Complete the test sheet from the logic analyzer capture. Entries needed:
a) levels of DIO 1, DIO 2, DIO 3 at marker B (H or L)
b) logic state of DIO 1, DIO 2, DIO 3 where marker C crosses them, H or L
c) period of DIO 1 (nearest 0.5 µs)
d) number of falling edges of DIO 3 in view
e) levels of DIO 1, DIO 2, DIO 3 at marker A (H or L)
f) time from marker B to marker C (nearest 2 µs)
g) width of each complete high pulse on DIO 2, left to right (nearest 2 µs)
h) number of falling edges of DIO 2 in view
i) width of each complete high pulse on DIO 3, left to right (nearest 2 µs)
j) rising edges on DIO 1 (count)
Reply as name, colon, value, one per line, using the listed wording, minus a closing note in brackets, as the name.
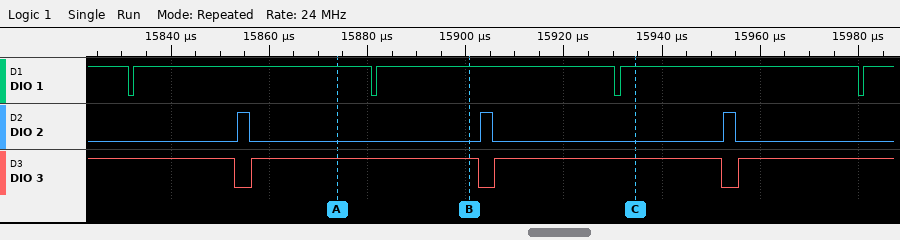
levels of DIO 1, DIO 2, DIO 3 at marker B: DIO 1=H, DIO 2=L, DIO 3=H
logic state of DIO 1, DIO 2, DIO 3 where marker C crosses them, H or L: DIO 1=H, DIO 2=L, DIO 3=H
period of DIO 1: 49.5 µs
number of falling edges of DIO 3 in view: 3
levels of DIO 1, DIO 2, DIO 3 at marker A: DIO 1=H, DIO 2=L, DIO 3=H
time from marker B to marker C: 34 µs
width of each complete high pulse on DIO 2, left to right: 2 µs, 2 µs, 2 µs
number of falling edges of DIO 2 in view: 3
width of each complete high pulse on DIO 3, left to right: 46 µs, 46 µs
rising edges on DIO 1: 4
